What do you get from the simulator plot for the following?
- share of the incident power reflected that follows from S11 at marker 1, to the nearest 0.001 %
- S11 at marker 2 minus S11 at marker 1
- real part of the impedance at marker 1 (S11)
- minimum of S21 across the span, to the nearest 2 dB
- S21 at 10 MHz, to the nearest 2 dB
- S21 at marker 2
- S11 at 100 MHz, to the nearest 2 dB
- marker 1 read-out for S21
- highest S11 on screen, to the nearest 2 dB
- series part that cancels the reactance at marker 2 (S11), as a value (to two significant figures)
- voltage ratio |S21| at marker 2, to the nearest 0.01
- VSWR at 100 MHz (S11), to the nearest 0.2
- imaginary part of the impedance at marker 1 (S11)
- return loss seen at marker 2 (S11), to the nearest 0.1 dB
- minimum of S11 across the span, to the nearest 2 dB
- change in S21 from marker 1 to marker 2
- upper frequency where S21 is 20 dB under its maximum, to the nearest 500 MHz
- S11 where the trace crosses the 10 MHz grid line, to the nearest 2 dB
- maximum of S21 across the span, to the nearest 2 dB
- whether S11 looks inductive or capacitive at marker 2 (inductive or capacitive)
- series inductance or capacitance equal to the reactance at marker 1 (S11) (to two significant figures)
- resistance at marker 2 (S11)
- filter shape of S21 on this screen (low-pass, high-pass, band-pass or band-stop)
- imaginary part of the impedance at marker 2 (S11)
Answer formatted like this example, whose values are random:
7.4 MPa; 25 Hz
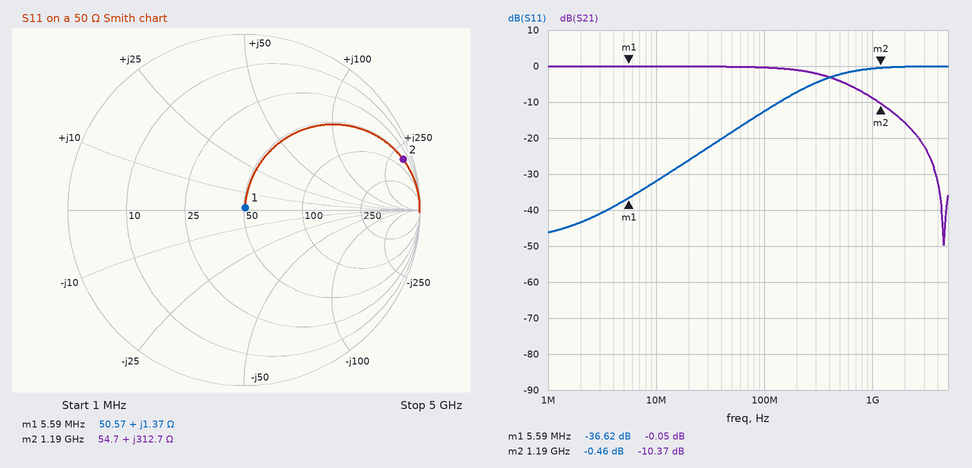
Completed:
0.022 %; 36.16 dB; 50.57 Ω; -50 dB; 0 dB; -10.37 dB; -12 dB; -0.05 dB; 0 dB; 430 fF; 0.30; 1.6; +1.37 Ω; 0.5 dB; -46 dB; -10.32 dB; 2.5 GHz; -32 dB; 0 dB; inductive; 39 nH; 54.7 Ω; low-pass; +312.7 Ω
